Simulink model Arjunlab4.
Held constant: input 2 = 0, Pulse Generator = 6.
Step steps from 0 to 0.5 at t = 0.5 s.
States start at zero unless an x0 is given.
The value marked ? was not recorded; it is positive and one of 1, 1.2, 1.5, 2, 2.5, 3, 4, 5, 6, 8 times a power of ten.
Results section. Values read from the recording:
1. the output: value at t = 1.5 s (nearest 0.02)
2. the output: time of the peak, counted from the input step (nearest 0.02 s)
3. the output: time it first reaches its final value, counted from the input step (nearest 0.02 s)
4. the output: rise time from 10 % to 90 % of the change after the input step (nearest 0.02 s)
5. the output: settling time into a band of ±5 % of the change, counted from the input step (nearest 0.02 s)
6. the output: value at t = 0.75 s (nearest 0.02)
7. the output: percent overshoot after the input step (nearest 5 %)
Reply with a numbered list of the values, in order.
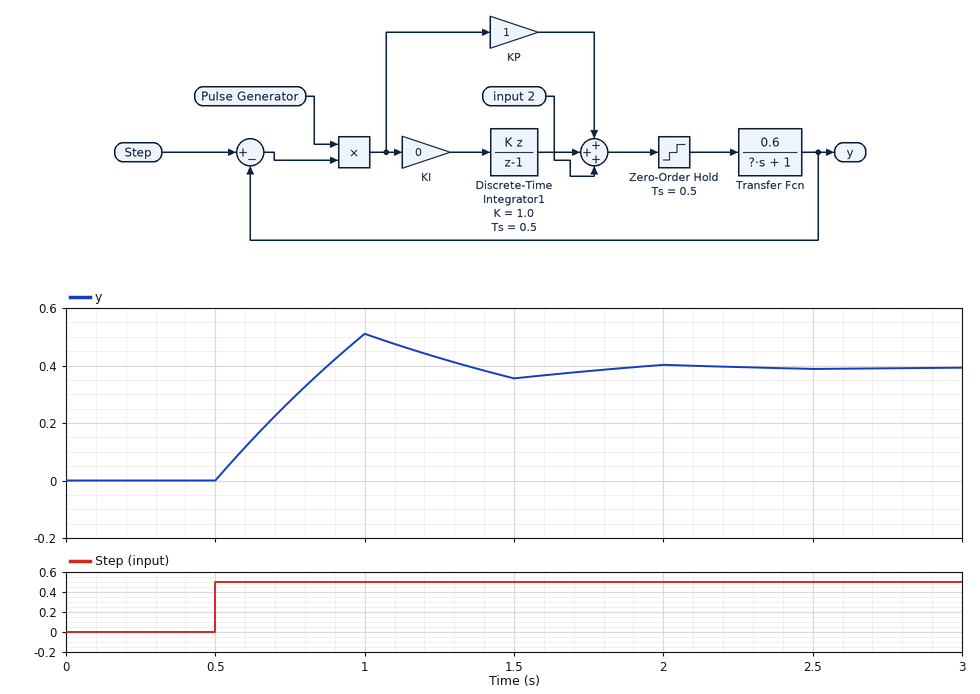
1. 0.36
2. 0.50 s
3. 0.36 s
4. 0.30 s
5. 1.16 s
6. 0.28
7. 30 %
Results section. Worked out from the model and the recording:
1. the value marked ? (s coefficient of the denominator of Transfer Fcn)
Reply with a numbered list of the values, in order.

1. 1.5
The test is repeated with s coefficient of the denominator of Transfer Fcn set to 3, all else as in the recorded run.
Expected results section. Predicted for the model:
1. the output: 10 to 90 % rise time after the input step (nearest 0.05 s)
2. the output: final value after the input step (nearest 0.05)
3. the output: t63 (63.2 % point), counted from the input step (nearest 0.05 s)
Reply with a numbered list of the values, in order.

1. 0.90 s
2. 0.40
3. 0.45 s
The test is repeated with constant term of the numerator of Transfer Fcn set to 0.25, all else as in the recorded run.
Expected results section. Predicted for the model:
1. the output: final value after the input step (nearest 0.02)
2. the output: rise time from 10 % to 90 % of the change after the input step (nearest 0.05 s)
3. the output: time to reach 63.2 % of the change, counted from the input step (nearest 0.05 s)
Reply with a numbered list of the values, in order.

1. 0.30
2. 0.90 s
3. 0.45 s
